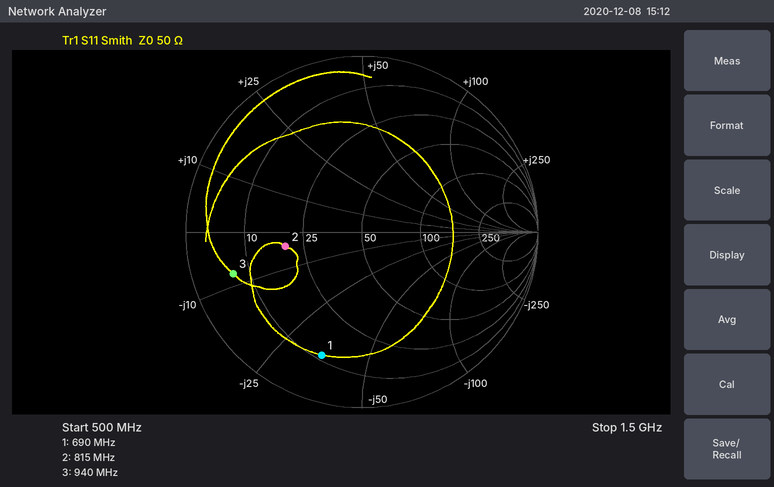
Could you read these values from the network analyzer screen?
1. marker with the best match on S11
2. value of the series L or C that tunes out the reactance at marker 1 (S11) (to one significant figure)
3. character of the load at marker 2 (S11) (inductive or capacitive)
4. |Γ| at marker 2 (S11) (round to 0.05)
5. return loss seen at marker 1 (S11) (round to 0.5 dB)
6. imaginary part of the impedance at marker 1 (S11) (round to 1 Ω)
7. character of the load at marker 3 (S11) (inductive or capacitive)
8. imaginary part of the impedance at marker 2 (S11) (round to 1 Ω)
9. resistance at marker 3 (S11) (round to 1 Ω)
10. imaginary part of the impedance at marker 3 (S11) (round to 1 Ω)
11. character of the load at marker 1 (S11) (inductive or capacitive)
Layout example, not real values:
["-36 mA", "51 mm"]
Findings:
["marker 2", "8 nH", "capacitive", "0.45", "2.5 dB", "-35 Ω", "capacitive", "-4 Ω", "7 Ω", "-8 Ω", "capacitive"]
